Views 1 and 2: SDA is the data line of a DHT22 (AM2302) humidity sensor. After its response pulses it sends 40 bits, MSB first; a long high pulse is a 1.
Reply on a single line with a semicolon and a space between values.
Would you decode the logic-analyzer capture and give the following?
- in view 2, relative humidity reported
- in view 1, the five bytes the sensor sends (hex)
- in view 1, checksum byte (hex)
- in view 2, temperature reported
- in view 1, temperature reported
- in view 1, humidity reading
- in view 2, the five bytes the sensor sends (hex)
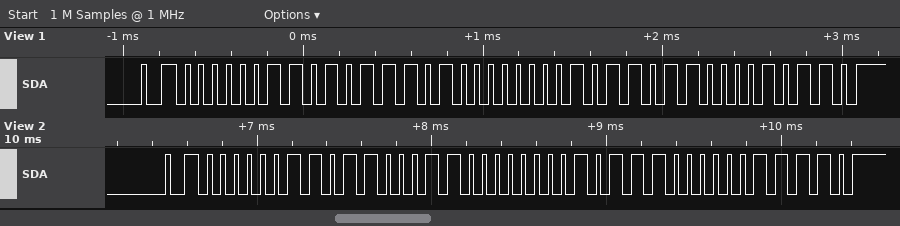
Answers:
86.7 %; 03 5D 00 B6 16; 0x16; 18.4 °C; 18.2 °C; 86.1 %; 03 63 00 B8 1E
